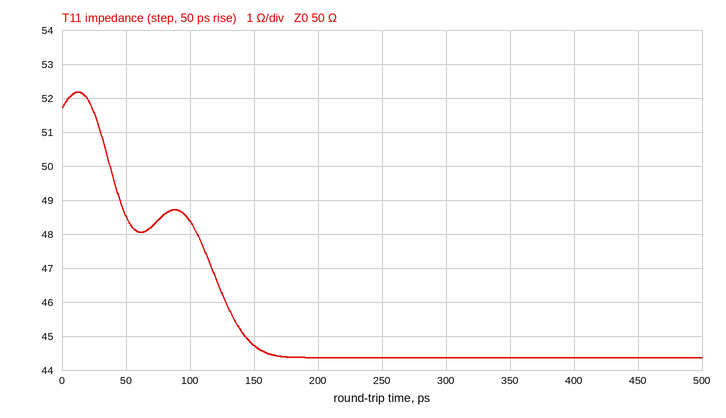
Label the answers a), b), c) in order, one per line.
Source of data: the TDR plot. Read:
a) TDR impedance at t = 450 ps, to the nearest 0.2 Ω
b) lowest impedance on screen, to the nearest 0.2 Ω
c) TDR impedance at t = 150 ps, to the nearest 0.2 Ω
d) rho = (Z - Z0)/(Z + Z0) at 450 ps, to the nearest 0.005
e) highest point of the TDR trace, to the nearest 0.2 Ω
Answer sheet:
a) 44.4 Ω
b) 44.4 Ω
c) 44.8 Ω
d) -0.060
e) 52.2 Ω
